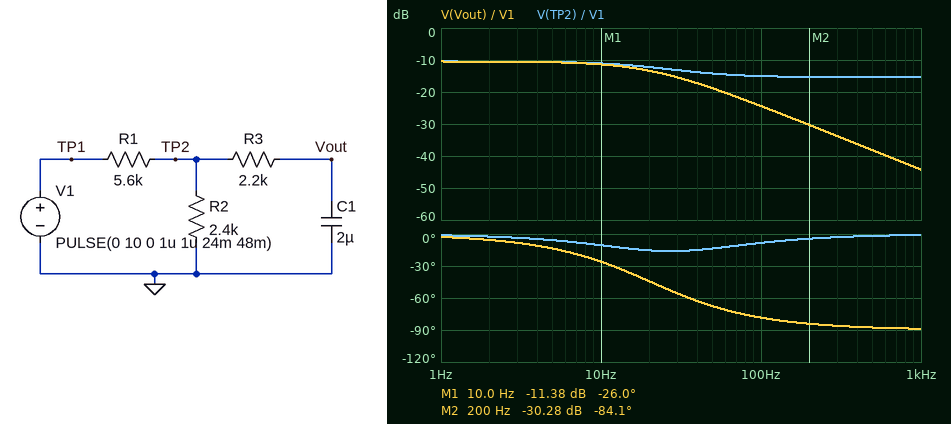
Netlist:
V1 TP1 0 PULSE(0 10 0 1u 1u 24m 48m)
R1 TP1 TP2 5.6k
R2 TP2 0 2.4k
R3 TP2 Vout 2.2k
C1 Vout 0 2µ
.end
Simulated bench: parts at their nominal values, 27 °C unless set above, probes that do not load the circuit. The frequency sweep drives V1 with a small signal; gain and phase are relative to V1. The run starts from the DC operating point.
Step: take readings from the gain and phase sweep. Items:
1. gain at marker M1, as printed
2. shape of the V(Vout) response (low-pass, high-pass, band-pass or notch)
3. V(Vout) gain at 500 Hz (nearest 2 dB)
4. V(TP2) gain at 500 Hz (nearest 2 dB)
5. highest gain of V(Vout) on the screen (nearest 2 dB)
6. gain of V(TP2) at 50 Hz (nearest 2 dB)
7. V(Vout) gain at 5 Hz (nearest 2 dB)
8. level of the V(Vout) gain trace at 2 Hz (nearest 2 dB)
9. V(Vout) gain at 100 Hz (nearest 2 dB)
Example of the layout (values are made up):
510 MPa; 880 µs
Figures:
-11.38 dB; low-pass; -38 dB; -16 dB; -10 dB; -14 dB; -10 dB; -10 dB; -24 dB
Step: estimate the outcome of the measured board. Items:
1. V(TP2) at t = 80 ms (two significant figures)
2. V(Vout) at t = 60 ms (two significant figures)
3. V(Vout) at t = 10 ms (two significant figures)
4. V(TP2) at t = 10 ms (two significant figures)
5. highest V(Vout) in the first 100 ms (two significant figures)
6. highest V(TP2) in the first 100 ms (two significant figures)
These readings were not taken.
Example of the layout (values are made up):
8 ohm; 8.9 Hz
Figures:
440 mV; 2.4 V; 2.2 V; 2.6 V; 2.9 V; 2.9 V
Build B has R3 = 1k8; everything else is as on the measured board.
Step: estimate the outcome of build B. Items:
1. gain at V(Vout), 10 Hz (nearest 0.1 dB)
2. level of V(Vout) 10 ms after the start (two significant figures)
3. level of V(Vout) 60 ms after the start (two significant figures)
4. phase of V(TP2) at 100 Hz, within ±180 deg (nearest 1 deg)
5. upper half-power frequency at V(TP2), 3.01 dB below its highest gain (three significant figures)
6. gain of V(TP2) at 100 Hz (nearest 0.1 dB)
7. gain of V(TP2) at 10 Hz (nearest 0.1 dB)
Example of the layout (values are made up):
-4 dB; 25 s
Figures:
-11.2 dB; 2.3 V; 2.5 V; -11 deg; 33.5 Hz; -15.6 dB; -11.0 dB
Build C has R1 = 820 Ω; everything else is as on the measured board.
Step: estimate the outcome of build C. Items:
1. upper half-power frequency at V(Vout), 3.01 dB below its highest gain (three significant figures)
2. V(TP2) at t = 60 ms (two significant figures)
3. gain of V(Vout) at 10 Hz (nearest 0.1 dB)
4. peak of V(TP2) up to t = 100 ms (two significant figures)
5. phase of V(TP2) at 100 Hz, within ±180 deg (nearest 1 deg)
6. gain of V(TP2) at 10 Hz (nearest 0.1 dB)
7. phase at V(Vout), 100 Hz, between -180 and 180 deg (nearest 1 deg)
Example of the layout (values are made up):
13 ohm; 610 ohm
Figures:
28.3 Hz; 7.3 V; -3.1 dB; 7.4 V; -4 deg; -2.7 dB; -74 deg
